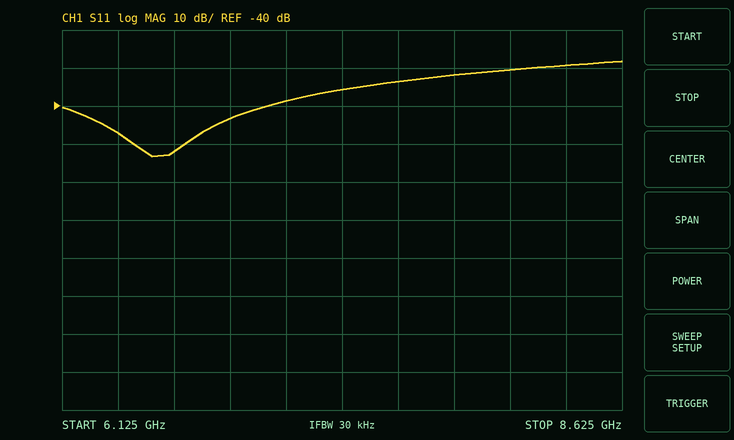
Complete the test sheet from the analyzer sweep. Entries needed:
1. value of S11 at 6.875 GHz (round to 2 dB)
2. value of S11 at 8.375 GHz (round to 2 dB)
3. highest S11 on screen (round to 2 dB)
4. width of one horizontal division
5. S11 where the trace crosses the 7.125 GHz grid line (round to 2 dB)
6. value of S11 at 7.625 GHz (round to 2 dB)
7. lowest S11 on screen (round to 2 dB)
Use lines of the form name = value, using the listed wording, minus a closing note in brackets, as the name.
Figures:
value of S11 at 6.875 GHz = -44 dB
value of S11 at 8.375 GHz = -30 dB
highest S11 on screen = -28 dB
width of one horizontal division = 250 MHz
S11 where the trace crosses the 7.125 GHz grid line = -38 dB
value of S11 at 7.625 GHz = -34 dB
lowest S11 on screen = -54 dB
